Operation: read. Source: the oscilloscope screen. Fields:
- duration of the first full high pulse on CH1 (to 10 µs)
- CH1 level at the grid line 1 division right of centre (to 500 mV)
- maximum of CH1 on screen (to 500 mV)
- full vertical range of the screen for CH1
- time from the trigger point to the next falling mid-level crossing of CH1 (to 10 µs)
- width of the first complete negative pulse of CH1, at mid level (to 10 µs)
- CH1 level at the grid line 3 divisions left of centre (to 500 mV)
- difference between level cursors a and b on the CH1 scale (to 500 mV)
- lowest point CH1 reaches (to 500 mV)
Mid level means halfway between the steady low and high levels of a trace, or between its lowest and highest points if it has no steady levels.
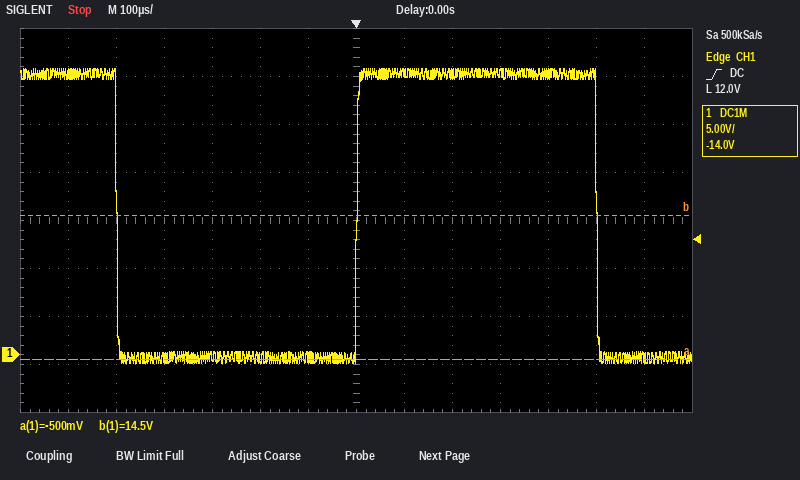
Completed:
500 µs
29.5 V
30.0 V
40 V
500 µs
500 µs
0.0 V
15.0 V
-1.0 V
